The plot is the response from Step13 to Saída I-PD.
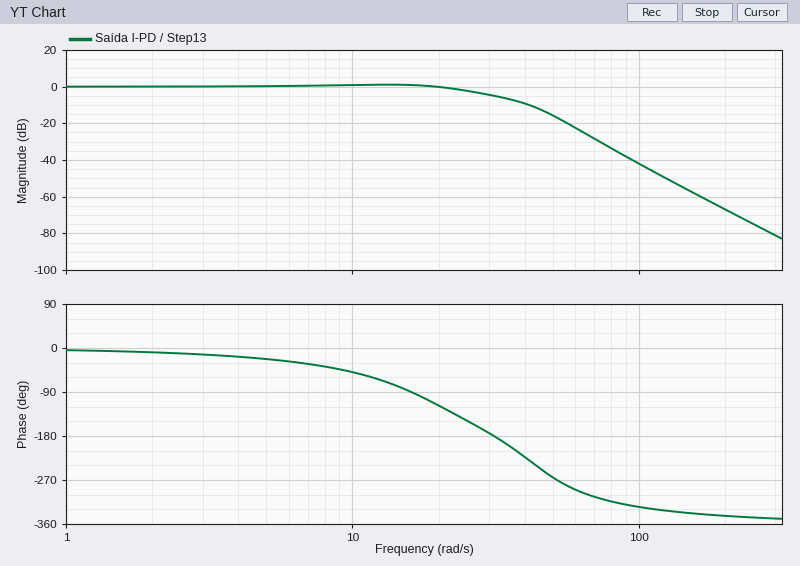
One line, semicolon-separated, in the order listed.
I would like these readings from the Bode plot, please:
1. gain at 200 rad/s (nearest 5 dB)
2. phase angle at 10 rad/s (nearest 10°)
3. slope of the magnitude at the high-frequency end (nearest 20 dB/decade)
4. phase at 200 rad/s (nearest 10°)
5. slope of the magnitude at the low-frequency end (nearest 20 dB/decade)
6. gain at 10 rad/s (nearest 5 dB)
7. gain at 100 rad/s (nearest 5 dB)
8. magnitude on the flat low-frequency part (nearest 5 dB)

-65 dB; -50°; -80 dB/decade; -340°; 0 dB/decade; 0 dB; -40 dB; 0 dB
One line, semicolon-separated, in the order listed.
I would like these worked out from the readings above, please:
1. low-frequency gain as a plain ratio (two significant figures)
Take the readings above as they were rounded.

1.0
